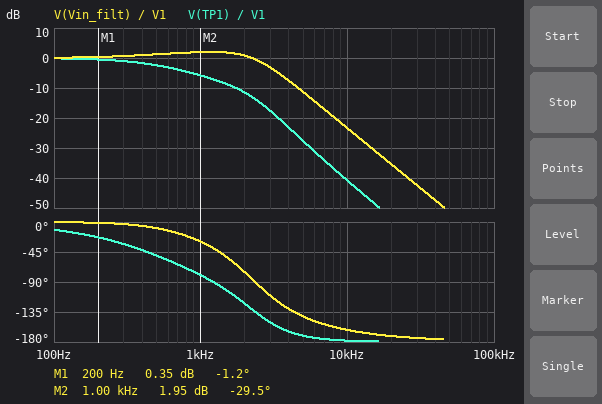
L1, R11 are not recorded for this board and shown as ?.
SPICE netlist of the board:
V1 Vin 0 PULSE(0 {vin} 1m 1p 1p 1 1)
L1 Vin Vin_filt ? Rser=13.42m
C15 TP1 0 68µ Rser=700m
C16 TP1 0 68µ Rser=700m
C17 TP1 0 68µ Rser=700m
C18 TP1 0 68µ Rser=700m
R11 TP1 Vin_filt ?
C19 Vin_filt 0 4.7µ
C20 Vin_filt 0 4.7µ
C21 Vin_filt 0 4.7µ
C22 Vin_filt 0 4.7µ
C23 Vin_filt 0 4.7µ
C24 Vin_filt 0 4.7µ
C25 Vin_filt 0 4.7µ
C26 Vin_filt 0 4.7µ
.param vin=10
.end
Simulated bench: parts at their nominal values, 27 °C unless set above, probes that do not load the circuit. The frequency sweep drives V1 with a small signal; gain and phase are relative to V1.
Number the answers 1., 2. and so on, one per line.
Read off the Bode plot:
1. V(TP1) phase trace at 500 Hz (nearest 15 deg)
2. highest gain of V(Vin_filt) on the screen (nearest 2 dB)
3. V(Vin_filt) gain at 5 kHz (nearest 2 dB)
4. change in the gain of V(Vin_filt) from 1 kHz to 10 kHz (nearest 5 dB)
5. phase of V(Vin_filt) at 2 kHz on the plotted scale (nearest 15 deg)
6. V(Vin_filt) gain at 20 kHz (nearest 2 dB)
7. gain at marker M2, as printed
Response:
1. -45 deg
2. 2 dB
3. -12 dB
4. -25 dB
5. -75 deg
6. -36 dB
7. 1.95 dB
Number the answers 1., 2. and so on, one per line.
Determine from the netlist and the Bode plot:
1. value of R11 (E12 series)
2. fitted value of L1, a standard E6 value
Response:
1. 1.2 Ω
2. 100 µH
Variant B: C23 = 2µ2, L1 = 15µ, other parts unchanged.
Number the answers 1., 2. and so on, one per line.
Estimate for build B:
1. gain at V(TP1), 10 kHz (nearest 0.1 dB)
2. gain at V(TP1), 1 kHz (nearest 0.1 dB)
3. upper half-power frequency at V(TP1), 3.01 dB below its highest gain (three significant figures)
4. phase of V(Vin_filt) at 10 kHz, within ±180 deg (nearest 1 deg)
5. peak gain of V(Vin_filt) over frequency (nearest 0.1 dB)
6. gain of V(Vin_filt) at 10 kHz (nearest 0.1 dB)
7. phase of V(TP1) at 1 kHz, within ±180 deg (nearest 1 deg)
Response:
1. -19.8 dB
2. -7.5 dB
3. 445 Hz
4. -147 deg
5. 6.5 dB
6. -2.3 dB
7. -54 deg
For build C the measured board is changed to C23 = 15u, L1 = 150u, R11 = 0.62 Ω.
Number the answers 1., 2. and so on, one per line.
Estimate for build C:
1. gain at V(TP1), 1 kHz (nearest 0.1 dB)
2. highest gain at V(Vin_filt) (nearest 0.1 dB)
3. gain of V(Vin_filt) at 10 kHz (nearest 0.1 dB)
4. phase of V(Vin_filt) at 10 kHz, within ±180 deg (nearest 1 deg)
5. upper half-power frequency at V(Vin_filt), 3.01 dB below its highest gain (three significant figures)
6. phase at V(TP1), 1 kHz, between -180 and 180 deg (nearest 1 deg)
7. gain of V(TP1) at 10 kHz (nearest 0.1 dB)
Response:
1. -2.2 dB
2. 4.3 dB
3. -29.7 dB
4. -157 deg
5. 1.06 kHz
6. -115 deg
7. -42.4 dB
